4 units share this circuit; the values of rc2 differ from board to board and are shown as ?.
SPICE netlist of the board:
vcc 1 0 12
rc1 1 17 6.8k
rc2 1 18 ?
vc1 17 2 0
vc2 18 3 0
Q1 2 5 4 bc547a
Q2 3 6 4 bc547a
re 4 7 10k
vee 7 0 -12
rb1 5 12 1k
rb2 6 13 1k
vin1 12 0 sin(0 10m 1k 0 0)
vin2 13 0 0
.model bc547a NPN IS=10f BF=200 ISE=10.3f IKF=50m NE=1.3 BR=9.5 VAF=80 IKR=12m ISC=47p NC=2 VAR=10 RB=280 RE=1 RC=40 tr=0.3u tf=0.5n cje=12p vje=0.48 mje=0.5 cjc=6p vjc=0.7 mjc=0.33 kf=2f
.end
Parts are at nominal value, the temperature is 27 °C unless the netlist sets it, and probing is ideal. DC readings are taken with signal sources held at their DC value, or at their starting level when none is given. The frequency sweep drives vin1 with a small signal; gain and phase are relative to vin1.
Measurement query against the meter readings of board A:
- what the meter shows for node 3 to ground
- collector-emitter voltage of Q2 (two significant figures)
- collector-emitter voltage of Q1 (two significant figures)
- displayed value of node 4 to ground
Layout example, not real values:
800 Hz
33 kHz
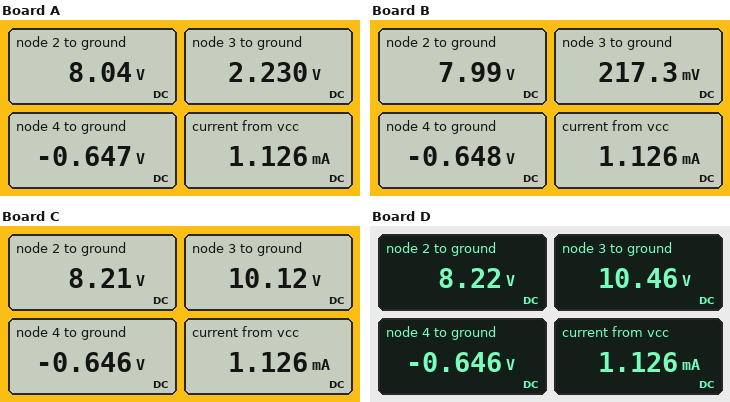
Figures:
2.230 V
2.9 V
8.7 V
-0.647 V
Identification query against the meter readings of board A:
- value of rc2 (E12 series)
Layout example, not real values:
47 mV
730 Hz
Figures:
18 kΩ
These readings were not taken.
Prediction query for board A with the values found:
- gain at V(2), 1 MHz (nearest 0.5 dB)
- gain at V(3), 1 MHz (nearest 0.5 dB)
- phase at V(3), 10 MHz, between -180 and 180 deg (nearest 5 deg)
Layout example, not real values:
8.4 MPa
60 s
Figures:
20.0 dB
27.0 dB
-95 deg
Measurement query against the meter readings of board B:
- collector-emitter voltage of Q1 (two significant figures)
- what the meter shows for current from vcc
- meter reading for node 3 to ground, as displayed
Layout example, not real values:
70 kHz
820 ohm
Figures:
8.6 V
1.126 mA
217.3 mV
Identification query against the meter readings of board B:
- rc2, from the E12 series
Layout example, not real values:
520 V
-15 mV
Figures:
22 kΩ
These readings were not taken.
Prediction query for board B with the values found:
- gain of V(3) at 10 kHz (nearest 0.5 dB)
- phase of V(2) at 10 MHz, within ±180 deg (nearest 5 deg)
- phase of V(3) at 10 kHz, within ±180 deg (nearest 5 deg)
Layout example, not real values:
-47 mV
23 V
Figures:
44.5 dB
90 deg
-5 deg
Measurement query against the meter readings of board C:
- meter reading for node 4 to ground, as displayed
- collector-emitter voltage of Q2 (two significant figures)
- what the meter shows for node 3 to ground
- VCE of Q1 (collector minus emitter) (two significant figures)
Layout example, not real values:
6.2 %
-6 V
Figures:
-0.646 V
11 V
10.12 V
8.9 V
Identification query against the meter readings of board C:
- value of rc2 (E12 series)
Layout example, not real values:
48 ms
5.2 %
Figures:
3.3 kΩ
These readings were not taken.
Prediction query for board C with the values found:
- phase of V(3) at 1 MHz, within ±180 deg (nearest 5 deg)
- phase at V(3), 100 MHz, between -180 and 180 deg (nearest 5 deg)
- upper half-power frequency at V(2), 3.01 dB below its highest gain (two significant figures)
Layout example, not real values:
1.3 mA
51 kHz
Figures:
-65 deg
-10 deg
470 kHz
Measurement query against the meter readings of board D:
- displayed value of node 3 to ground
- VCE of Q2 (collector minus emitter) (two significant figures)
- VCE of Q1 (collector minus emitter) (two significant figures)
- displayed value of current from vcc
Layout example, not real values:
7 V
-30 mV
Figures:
10.46 V
11 V
8.9 V
1.126 mA
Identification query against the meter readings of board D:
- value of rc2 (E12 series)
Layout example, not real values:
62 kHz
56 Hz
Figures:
2.7 kΩ
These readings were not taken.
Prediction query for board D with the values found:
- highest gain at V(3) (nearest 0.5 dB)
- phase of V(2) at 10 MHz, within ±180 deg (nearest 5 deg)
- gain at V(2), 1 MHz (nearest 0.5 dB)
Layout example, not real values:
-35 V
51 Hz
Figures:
27.0 dB
75 deg
28.0 dB
